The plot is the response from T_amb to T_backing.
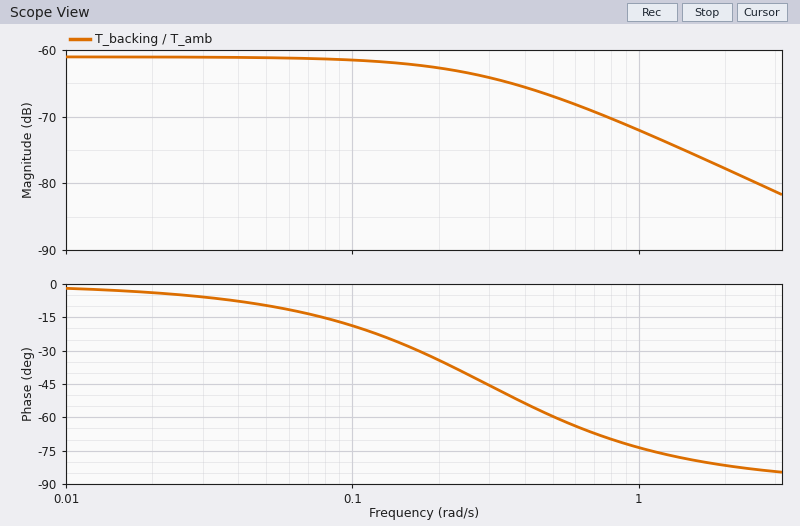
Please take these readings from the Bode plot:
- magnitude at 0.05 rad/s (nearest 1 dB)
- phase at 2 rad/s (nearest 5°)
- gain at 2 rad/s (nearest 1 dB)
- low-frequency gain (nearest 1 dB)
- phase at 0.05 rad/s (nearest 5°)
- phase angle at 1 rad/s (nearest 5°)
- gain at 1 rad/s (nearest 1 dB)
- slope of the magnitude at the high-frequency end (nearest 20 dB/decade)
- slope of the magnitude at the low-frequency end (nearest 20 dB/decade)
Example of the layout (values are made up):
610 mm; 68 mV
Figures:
-61 dB; -80°; -78 dB; -61 dB; -10°; -75°; -72 dB; -20 dB/decade; 0 dB/decade
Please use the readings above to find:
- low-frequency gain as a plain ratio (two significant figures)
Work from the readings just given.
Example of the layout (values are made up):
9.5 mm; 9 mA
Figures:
0.00089
